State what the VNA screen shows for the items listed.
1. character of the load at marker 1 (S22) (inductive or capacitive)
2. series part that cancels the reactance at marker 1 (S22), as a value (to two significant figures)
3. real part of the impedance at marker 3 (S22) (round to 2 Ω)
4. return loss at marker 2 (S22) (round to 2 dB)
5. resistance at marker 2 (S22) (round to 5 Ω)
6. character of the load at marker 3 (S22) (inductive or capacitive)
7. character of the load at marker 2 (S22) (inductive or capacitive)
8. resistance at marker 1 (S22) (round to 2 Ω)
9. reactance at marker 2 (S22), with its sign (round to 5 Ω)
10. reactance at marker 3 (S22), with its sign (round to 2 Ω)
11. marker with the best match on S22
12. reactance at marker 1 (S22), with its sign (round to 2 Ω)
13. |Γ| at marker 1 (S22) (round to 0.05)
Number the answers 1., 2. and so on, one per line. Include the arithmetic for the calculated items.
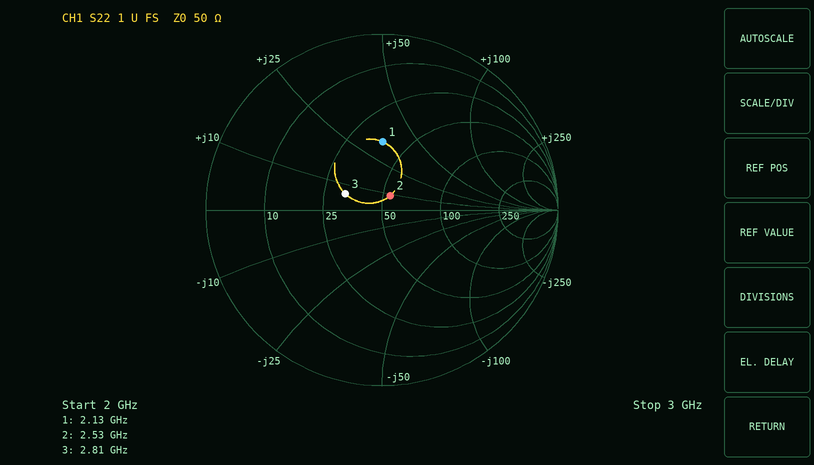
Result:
1. inductive
2. C = 1/(2π × 2.13 GHz × 34 Ω) ≈ 2.2 pF
3. 32 Ω
4. 20 dB
5. 55 Ω
6. inductive
7. inductive
8. 38 Ω
9. +10 Ω
10. +6 Ω
11. marker 2
12. +34 Ω
13. 0.40
